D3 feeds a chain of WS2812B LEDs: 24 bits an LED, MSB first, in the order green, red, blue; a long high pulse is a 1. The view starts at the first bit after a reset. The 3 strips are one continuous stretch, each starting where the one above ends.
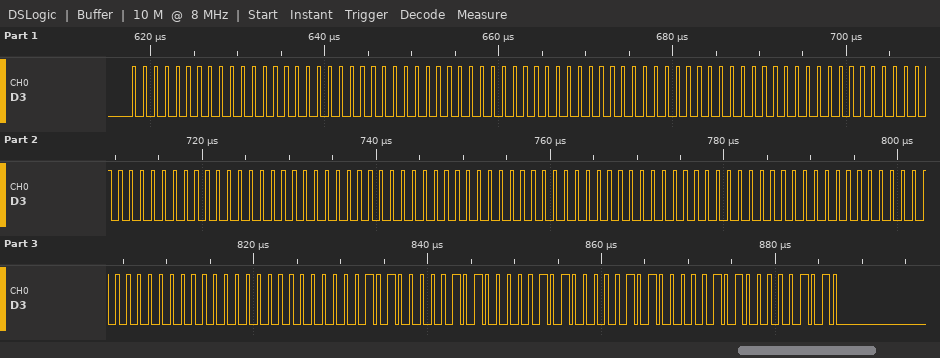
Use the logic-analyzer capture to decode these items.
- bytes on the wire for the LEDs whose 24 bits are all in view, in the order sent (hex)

00 00 00 00 00 00 00 00 00 00 00 00 00 00 00 00 00 00 00 00 00 0A 0A 0A 0A 0A 0A
